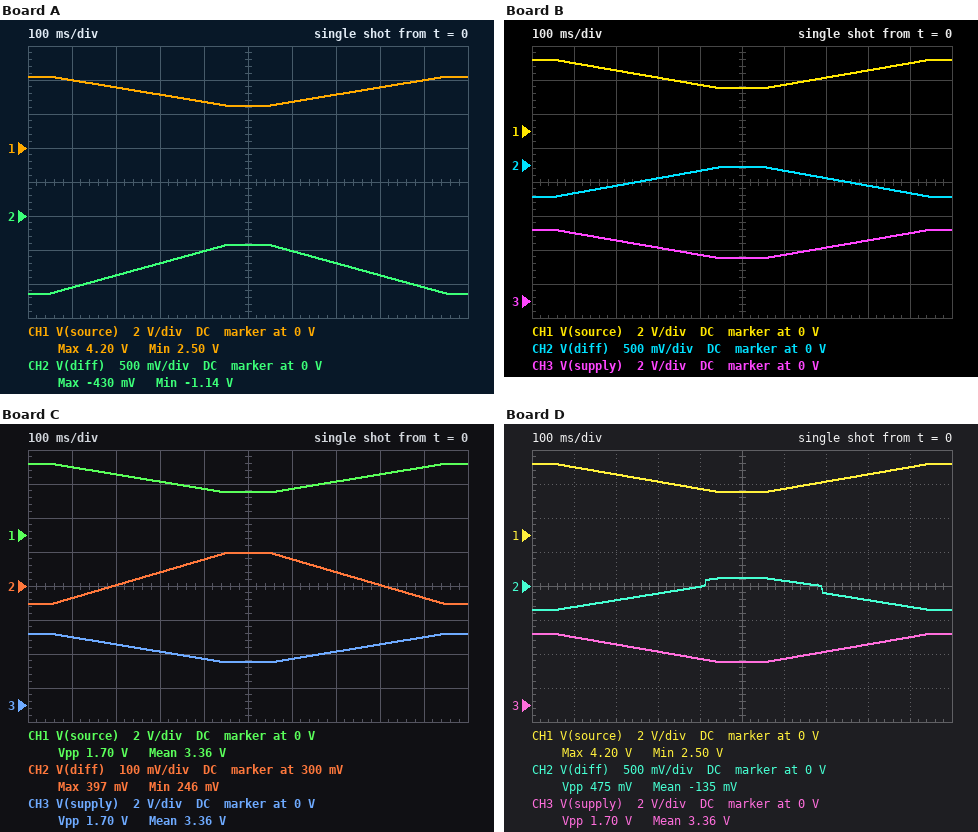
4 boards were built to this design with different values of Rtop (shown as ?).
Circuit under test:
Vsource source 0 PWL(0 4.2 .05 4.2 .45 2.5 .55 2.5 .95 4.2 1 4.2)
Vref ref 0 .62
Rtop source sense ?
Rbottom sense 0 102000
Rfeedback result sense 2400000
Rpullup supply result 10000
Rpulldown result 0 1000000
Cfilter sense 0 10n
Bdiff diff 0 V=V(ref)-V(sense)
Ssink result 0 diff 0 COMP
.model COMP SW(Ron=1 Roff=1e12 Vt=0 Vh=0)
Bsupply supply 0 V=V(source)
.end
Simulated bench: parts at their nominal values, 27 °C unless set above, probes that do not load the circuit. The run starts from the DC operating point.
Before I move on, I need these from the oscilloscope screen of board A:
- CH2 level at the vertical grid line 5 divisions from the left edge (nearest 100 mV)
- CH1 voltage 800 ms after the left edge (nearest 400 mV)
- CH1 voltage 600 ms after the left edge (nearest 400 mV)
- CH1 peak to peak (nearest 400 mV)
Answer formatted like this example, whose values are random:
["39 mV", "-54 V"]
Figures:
["-400 mV", "3.6 V", "2.8 V", "1.6 V"]
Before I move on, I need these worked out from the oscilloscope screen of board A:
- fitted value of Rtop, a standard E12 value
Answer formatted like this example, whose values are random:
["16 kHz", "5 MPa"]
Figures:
["150 kΩ"]
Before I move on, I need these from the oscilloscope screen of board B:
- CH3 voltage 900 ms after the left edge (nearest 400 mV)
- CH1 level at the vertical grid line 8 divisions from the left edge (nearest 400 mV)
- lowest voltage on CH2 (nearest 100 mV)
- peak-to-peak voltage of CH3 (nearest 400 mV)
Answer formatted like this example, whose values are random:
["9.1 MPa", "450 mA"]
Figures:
["4.0 V", "3.6 V", "-500 mV", "1.6 V"]
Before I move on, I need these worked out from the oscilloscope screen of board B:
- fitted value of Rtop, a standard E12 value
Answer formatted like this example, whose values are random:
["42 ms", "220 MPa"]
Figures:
["330 kΩ"]
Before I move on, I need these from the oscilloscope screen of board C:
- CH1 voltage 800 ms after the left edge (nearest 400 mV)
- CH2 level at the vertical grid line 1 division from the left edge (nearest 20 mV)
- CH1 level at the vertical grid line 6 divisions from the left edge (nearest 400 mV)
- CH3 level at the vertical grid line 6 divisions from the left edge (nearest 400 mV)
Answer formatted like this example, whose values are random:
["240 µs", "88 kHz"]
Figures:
["3.6 V", "260 mV", "2.8 V", "2.8 V"]
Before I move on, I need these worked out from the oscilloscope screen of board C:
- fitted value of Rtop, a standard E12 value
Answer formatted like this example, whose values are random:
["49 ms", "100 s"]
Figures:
["1 MΩ"]
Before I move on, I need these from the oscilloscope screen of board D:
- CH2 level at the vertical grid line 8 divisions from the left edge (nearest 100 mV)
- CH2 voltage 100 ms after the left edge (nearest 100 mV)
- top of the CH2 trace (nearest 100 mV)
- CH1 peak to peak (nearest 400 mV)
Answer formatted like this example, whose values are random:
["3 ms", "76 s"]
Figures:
["-200 mV", "-300 mV", "100 mV", "1.6 V"]
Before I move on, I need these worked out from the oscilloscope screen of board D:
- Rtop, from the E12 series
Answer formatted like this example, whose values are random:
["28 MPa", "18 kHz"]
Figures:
["390 kΩ"]
